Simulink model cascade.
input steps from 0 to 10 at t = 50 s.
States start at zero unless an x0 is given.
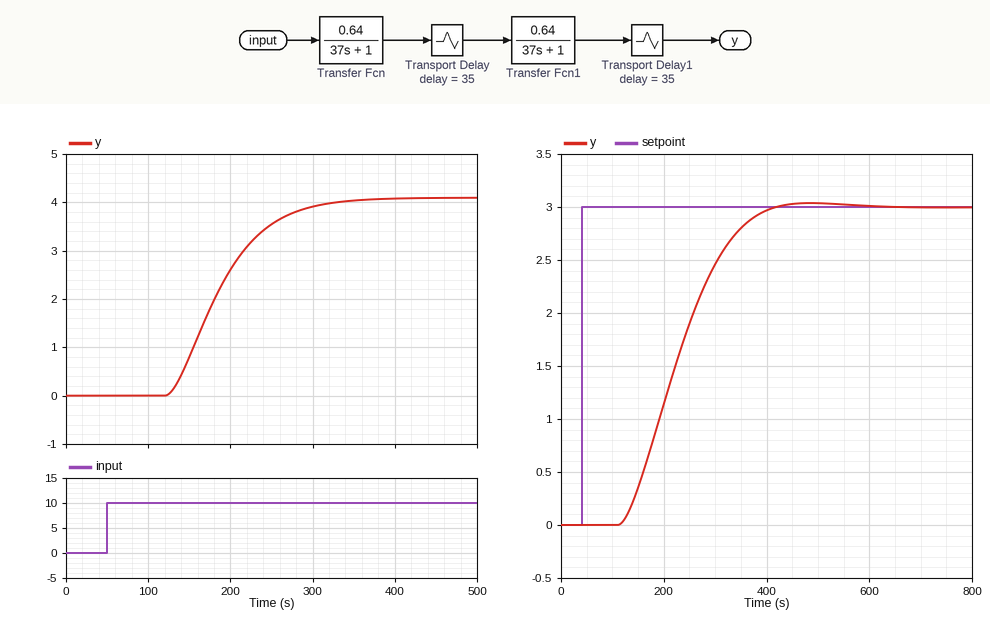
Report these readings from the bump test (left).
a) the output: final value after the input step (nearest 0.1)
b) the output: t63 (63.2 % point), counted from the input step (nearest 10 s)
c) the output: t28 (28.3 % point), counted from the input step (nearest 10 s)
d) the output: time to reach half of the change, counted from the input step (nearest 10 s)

4.1
150 s
110 s
130 s
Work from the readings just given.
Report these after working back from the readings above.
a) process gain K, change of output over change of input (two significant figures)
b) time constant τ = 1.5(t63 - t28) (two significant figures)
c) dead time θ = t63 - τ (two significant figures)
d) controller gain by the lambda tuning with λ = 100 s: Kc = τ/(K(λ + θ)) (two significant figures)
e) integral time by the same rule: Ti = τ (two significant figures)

0.41
60 s
90 s
0.77
60 s
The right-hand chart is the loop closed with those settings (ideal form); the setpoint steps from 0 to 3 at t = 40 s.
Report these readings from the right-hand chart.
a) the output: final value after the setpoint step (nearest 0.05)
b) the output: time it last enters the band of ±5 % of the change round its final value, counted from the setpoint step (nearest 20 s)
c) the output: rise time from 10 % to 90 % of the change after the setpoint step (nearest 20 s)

3.00
320 s
180 s
